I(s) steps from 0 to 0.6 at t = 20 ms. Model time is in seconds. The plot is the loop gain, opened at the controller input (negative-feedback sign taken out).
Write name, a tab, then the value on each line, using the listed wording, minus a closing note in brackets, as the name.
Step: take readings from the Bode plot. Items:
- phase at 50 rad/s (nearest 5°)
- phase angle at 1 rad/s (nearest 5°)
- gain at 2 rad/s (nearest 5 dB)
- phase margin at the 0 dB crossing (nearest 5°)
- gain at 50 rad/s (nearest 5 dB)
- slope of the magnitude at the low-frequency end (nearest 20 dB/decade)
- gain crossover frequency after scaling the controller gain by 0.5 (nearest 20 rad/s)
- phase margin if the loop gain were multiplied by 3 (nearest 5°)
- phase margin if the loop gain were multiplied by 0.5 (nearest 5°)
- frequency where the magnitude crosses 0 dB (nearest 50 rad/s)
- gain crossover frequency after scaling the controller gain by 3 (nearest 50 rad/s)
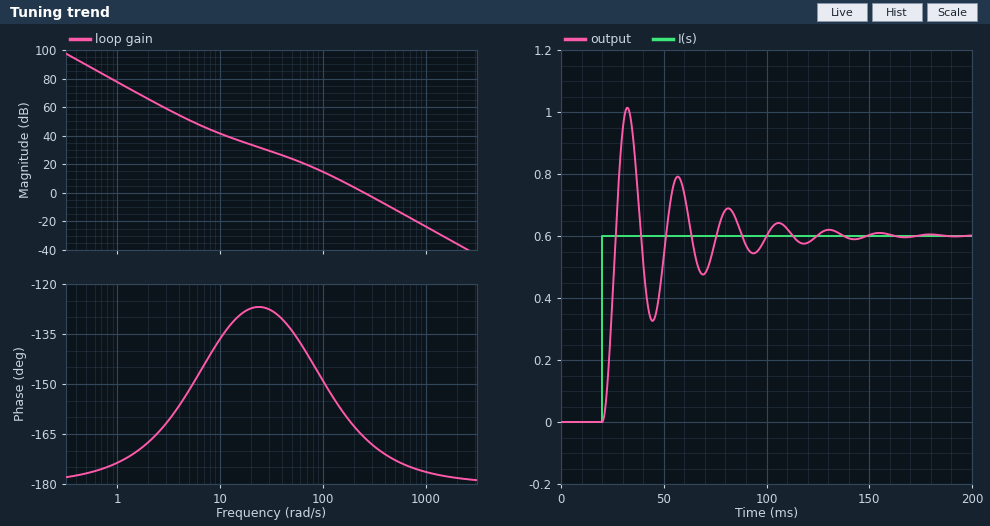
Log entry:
phase at 50 rad/s	-135°
phase angle at 1 rad/s	-175°
gain at 2 rad/s	65 dB
phase margin at the 0 dB crossing	15°
gain at 50 rad/s	25 dB
slope of the magnitude at the low-frequency end	-40 dB/decade
gain crossover frequency after scaling the controller gain by 0.5	180 rad/s
phase margin if the loop gain were multiplied by 3	10°
phase margin if the loop gain were multiplied by 0.5	20°
frequency where the magnitude crosses 0 dB	250 rad/s
gain crossover frequency after scaling the controller gain by 3	450 rad/s
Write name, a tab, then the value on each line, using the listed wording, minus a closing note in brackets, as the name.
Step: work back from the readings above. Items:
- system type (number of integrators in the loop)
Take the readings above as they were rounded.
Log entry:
system type	2
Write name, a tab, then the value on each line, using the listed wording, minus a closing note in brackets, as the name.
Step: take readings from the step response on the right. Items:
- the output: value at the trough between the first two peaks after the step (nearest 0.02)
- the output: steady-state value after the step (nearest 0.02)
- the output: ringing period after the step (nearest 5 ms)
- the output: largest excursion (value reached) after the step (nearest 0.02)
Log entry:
the output: value at the trough between the first two peaks after the step	0.32
the output: steady-state value after the step	0.60
the output: ringing period after the step	25 ms
the output: largest excursion (value reached) after the step	1.02
